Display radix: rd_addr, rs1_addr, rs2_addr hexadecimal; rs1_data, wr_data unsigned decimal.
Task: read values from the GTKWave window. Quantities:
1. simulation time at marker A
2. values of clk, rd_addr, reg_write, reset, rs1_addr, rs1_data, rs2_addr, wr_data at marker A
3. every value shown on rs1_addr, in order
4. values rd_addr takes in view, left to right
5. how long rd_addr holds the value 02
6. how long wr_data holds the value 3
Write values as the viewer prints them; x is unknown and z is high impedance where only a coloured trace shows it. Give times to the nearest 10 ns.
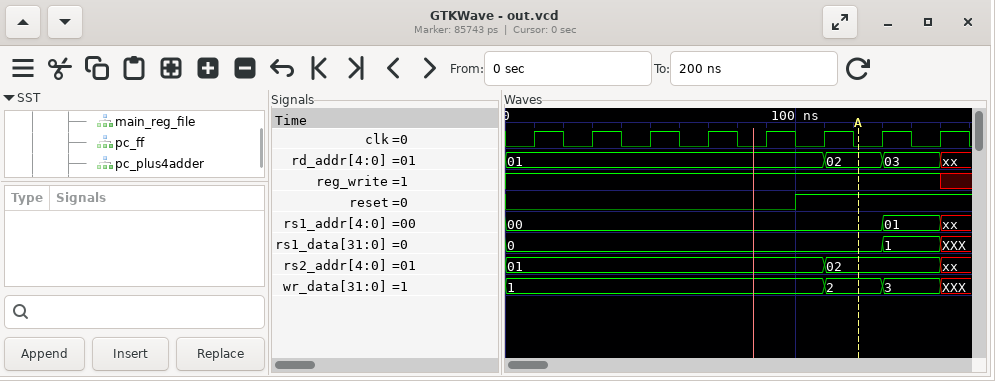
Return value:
120 ns
clk=0, rd_addr=02, reg_write=1, reset=1, rs1_addr=00, rs1_data=0, rs2_addr=02, wr_data=2
00, 01, xx
01, 02, 03, xx
20 ns
20 ns
